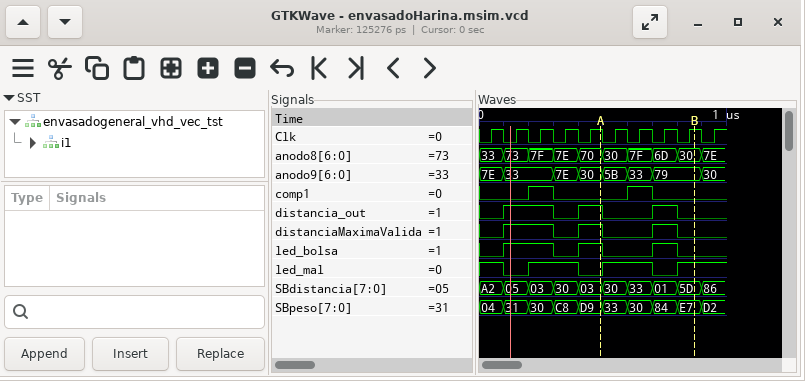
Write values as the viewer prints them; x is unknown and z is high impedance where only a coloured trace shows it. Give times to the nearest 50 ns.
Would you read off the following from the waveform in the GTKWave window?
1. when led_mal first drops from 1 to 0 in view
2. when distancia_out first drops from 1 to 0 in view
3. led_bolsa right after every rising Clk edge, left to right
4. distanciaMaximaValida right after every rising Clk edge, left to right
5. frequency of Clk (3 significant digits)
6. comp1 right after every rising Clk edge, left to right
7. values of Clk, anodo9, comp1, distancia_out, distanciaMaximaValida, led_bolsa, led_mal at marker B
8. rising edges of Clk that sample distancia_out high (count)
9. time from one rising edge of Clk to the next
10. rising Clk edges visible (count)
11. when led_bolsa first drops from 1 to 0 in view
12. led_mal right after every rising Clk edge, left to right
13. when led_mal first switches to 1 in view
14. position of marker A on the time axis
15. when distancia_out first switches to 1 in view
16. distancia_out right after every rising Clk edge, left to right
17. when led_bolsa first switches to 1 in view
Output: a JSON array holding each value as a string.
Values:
["100 ns", "300 ns", "0 1 1 0 1 0 0 1 0 0", "0 1 1 0 1 0 0 1 0 0", "10.0 MHz", "0 0 1 0 0 0 1 0 0 0", "Clk=1, anodo9=79, comp1=0, distancia_out=0, distanciaMaximaValida=0, led_bolsa=0, led_mal=1", "4", "100 ns", "10", "300 ns", "1 0 1 1 0 1 1 0 1 1", "200 ns", "500 ns", "100 ns", "0 1 1 0 1 0 0 1 0 0", "100 ns"]
